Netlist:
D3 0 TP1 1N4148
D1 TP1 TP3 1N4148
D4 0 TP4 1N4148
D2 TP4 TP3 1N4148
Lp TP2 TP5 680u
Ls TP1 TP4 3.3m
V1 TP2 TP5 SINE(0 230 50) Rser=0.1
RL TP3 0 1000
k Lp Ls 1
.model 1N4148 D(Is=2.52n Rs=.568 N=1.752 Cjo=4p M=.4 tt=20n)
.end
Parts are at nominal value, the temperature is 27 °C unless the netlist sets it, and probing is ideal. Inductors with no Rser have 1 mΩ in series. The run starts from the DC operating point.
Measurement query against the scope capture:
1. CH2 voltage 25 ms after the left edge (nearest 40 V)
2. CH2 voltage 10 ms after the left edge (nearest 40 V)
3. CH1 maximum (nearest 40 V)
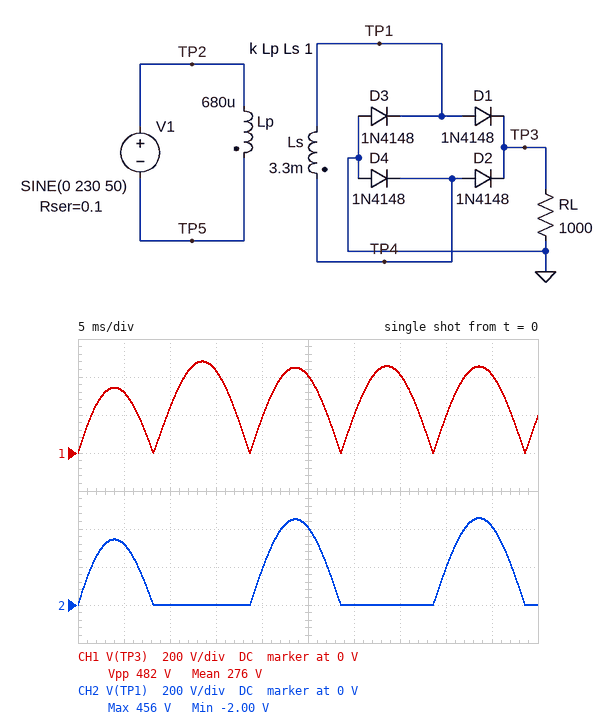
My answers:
400 V
0 V
480 V
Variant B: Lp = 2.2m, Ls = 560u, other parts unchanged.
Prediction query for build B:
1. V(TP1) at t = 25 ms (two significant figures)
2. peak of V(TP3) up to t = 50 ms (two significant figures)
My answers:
110 V
120 V
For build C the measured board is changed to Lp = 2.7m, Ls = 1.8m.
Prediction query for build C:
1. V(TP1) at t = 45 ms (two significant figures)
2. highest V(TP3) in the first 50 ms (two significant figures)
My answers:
180 V
200 V
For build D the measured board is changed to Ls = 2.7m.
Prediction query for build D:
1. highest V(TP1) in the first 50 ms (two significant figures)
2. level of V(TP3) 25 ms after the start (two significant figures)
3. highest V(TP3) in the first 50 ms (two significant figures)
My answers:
410 V
370 V
440 V
